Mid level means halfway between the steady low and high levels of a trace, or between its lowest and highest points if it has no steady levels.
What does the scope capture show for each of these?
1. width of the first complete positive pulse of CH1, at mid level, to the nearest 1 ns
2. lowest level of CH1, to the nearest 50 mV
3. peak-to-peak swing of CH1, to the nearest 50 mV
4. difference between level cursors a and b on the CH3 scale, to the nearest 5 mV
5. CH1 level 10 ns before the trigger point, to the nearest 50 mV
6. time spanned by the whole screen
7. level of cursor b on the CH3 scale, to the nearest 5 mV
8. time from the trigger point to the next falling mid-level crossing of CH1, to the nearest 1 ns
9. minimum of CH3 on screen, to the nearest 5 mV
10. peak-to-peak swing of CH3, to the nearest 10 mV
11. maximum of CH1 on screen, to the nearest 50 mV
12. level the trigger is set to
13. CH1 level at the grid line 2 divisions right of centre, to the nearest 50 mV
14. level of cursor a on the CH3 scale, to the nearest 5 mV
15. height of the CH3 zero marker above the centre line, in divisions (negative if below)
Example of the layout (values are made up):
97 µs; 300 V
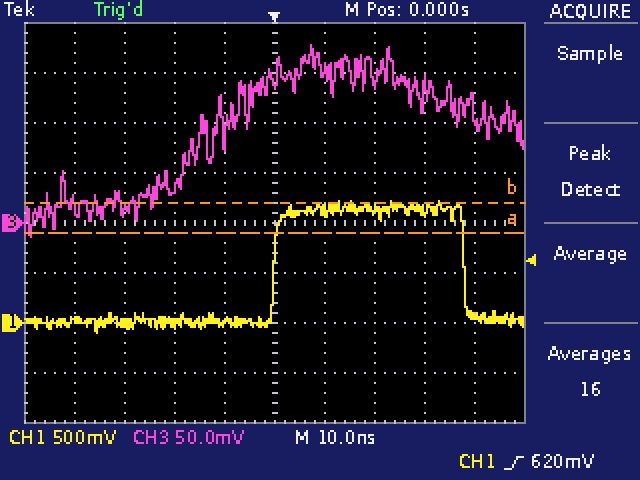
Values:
38 ns; -100 mV; 1.30 V; 30 mV; 0 mV; 100 ns; 20 mV; 38 ns; -15 mV; 190 mV; 1.20 V; 620 mV; 1.15 V; -10 mV; 0.0 div
